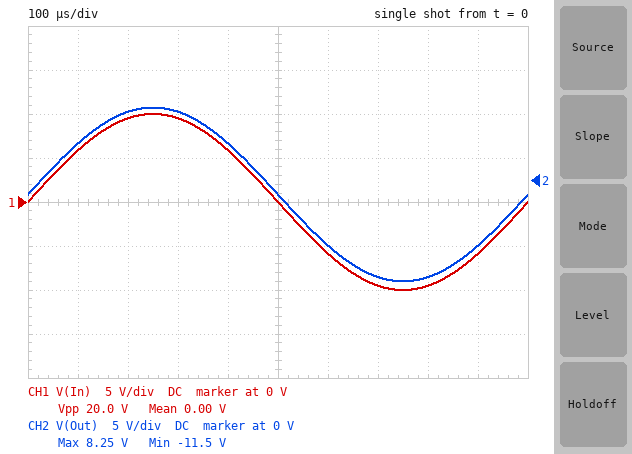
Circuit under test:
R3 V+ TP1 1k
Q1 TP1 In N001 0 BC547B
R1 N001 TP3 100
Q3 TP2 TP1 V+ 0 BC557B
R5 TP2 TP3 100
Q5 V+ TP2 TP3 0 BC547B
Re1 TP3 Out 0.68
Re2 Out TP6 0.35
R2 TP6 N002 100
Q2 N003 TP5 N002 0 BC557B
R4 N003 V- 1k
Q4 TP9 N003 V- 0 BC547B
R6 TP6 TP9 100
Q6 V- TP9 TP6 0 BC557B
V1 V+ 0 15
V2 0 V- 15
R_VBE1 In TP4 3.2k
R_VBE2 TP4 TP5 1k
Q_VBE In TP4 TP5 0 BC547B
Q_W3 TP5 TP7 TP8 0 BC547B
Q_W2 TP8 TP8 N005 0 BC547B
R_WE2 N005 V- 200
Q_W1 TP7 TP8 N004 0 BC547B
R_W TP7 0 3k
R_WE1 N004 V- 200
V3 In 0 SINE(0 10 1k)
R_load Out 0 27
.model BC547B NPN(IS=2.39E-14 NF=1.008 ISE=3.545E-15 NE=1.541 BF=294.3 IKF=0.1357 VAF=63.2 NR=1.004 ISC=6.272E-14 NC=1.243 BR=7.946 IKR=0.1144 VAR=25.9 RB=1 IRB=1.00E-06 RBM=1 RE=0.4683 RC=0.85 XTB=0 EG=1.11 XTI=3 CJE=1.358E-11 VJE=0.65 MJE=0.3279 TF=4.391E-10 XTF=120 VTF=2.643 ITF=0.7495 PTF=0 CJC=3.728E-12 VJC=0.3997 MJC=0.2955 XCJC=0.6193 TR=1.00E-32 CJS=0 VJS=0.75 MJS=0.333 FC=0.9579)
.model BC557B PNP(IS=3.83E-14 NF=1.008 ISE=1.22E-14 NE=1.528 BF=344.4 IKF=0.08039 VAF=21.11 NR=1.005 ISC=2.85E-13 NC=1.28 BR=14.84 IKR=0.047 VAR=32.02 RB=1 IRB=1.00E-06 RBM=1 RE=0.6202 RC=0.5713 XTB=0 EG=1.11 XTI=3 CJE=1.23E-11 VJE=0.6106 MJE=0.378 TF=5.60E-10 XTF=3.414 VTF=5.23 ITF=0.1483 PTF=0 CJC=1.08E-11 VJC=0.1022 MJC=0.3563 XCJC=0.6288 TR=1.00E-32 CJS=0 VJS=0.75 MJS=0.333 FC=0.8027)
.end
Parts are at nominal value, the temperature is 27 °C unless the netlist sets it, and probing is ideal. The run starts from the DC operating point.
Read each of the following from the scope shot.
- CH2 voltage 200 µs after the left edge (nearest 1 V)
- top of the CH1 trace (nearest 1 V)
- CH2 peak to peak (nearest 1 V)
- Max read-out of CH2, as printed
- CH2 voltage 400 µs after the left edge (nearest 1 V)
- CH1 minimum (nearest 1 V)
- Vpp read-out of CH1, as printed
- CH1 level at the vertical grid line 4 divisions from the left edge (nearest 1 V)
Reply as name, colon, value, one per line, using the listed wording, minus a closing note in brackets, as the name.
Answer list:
CH2 voltage 200 µs after the left edge: 8 V
top of the CH1 trace: 10 V
CH2 peak to peak: 20 V
Max read-out of CH2, as printed: 8.25 V
CH2 voltage 400 µs after the left edge: 4 V
CH1 minimum: -10 V
Vpp read-out of CH1, as printed: 20.0 V
CH1 level at the vertical grid line 4 divisions from the left edge: 6 V
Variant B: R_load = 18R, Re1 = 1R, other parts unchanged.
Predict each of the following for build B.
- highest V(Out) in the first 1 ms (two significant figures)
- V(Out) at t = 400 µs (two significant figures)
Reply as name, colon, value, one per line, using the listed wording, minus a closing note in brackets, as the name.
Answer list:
highest V(Out) in the first 1 ms: 8.1 V
V(Out) at t = 400 µs: 4.0 V
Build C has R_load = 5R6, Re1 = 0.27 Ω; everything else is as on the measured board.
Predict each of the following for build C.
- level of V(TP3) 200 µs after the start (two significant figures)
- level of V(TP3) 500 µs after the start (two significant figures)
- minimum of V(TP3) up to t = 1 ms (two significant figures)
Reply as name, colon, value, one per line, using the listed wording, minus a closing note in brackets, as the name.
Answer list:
level of V(TP3) 200 µs after the start: 8.6 V
level of V(TP3) 500 µs after the start: -750 mV
minimum of V(TP3) up to t = 1 ms: -11 V
